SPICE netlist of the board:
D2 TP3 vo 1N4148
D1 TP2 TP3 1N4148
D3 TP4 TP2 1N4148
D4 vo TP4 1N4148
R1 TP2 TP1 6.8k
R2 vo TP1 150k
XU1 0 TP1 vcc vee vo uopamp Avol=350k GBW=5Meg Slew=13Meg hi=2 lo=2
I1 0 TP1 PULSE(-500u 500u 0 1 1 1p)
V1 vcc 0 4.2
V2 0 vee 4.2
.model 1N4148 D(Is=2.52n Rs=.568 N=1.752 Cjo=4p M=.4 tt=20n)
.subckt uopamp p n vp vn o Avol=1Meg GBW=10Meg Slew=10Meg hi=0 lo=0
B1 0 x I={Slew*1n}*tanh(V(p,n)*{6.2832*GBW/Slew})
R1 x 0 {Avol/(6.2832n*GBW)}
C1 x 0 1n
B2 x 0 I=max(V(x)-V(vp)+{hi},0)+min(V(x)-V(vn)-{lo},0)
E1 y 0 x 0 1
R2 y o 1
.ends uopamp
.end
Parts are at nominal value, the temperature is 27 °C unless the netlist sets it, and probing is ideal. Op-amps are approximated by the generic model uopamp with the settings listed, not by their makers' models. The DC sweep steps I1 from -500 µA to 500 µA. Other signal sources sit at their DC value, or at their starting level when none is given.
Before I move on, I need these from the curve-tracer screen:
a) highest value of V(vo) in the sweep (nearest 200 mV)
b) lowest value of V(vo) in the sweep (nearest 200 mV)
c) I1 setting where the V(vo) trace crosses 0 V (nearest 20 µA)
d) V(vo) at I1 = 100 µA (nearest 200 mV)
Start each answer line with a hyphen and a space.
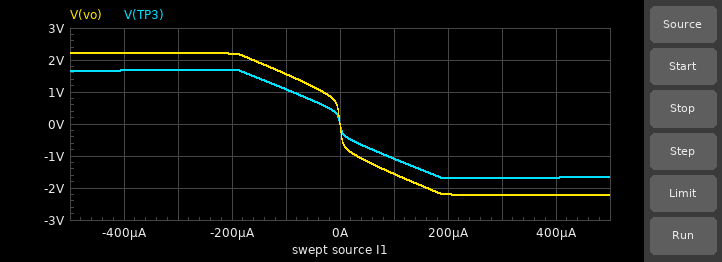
- 2.2 V
- -2.2 V
- 0 A
- -1.6 V
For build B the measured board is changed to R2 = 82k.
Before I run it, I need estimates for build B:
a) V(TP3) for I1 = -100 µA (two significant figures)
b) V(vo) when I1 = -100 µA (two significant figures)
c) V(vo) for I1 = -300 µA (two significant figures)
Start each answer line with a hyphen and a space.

- 1.0 V
- 1.5 V
- 2.2 V
